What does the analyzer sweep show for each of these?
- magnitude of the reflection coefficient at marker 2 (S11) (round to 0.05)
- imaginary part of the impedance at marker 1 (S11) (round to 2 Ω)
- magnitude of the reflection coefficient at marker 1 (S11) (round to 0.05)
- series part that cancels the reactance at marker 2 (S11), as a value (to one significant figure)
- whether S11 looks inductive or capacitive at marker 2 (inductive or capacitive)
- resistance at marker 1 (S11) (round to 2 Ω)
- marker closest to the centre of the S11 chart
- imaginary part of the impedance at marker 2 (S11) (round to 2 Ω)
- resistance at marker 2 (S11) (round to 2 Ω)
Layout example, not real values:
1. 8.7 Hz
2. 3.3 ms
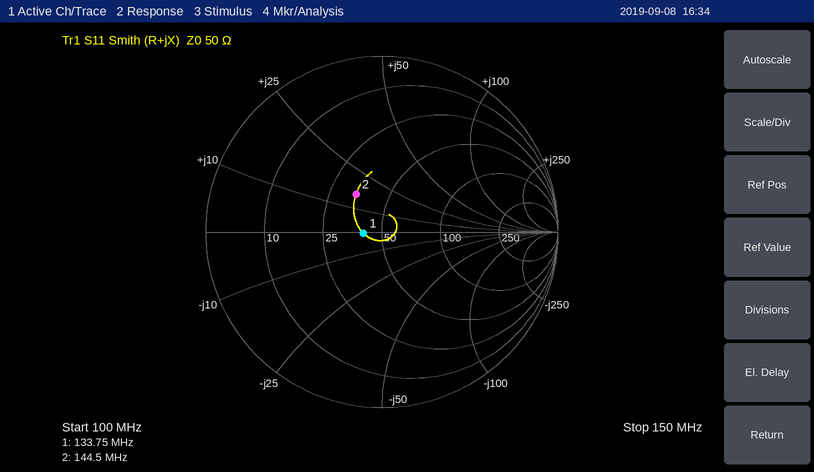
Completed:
1. 0.25
2. 0 Ω
3. 0.10
4. 70 pF
5. inductive
6. 40 Ω
7. marker 1
8. +16 Ω
9. 34 Ω
